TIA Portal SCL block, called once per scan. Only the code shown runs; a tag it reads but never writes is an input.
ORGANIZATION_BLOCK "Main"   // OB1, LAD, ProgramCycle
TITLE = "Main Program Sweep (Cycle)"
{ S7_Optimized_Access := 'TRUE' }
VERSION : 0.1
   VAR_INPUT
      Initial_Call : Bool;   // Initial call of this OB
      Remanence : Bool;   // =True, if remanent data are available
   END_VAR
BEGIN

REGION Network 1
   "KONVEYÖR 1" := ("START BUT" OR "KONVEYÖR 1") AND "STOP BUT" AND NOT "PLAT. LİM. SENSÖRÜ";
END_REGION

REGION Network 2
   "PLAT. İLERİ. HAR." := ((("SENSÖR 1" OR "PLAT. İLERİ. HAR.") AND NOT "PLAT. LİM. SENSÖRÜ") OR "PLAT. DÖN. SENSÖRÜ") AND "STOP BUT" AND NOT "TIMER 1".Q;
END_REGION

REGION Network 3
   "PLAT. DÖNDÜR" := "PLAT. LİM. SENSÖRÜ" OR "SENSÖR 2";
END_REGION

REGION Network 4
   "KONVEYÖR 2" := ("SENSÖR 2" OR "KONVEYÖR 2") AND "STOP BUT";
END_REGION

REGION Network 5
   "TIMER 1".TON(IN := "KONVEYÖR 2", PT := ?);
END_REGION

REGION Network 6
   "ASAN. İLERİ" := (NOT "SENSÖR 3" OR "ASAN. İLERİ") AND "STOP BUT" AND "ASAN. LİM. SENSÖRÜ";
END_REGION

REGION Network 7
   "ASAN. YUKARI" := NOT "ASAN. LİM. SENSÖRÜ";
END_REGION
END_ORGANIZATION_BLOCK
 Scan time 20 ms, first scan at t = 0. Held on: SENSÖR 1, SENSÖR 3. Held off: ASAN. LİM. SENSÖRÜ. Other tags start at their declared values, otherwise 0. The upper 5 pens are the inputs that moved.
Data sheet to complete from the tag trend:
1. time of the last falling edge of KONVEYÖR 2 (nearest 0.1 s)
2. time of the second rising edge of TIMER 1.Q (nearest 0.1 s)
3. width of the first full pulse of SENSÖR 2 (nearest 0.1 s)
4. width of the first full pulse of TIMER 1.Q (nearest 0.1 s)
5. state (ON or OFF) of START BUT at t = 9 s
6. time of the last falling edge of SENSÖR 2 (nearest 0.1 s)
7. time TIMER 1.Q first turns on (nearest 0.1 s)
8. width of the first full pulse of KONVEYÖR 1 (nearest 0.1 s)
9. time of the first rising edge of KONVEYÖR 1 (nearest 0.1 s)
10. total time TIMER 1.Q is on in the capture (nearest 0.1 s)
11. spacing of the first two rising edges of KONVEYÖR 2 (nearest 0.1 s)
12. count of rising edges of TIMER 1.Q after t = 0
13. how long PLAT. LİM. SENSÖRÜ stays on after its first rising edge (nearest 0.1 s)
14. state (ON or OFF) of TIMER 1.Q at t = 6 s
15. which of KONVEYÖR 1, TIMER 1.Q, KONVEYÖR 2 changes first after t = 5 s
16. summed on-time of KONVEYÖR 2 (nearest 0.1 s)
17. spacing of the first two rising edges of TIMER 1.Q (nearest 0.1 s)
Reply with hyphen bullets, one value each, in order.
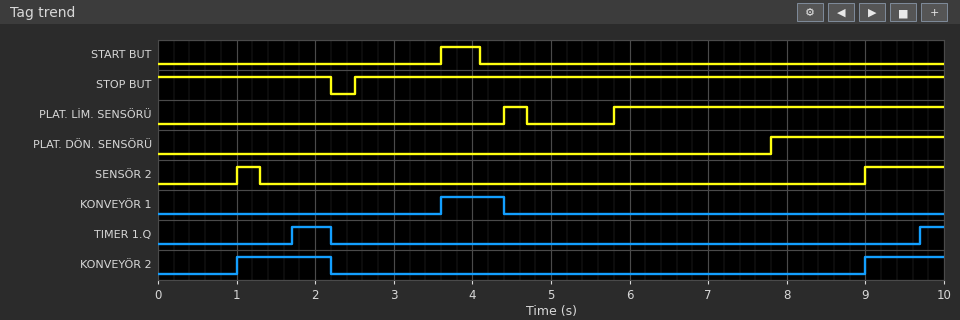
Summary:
- 2.2 s
- 9.7 s
- 0.3 s
- 0.5 s
- OFF
- 1.3 s
- 1.7 s
- 0.8 s
- 3.6 s
- 0.8 s
- 8.0 s
- 2
- 0.3 s
- OFF
- KONVEYÖR 2
- 2.2 s
- 8.0 s
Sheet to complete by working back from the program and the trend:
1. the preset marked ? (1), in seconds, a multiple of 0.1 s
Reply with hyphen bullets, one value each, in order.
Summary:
- 0.7 s
